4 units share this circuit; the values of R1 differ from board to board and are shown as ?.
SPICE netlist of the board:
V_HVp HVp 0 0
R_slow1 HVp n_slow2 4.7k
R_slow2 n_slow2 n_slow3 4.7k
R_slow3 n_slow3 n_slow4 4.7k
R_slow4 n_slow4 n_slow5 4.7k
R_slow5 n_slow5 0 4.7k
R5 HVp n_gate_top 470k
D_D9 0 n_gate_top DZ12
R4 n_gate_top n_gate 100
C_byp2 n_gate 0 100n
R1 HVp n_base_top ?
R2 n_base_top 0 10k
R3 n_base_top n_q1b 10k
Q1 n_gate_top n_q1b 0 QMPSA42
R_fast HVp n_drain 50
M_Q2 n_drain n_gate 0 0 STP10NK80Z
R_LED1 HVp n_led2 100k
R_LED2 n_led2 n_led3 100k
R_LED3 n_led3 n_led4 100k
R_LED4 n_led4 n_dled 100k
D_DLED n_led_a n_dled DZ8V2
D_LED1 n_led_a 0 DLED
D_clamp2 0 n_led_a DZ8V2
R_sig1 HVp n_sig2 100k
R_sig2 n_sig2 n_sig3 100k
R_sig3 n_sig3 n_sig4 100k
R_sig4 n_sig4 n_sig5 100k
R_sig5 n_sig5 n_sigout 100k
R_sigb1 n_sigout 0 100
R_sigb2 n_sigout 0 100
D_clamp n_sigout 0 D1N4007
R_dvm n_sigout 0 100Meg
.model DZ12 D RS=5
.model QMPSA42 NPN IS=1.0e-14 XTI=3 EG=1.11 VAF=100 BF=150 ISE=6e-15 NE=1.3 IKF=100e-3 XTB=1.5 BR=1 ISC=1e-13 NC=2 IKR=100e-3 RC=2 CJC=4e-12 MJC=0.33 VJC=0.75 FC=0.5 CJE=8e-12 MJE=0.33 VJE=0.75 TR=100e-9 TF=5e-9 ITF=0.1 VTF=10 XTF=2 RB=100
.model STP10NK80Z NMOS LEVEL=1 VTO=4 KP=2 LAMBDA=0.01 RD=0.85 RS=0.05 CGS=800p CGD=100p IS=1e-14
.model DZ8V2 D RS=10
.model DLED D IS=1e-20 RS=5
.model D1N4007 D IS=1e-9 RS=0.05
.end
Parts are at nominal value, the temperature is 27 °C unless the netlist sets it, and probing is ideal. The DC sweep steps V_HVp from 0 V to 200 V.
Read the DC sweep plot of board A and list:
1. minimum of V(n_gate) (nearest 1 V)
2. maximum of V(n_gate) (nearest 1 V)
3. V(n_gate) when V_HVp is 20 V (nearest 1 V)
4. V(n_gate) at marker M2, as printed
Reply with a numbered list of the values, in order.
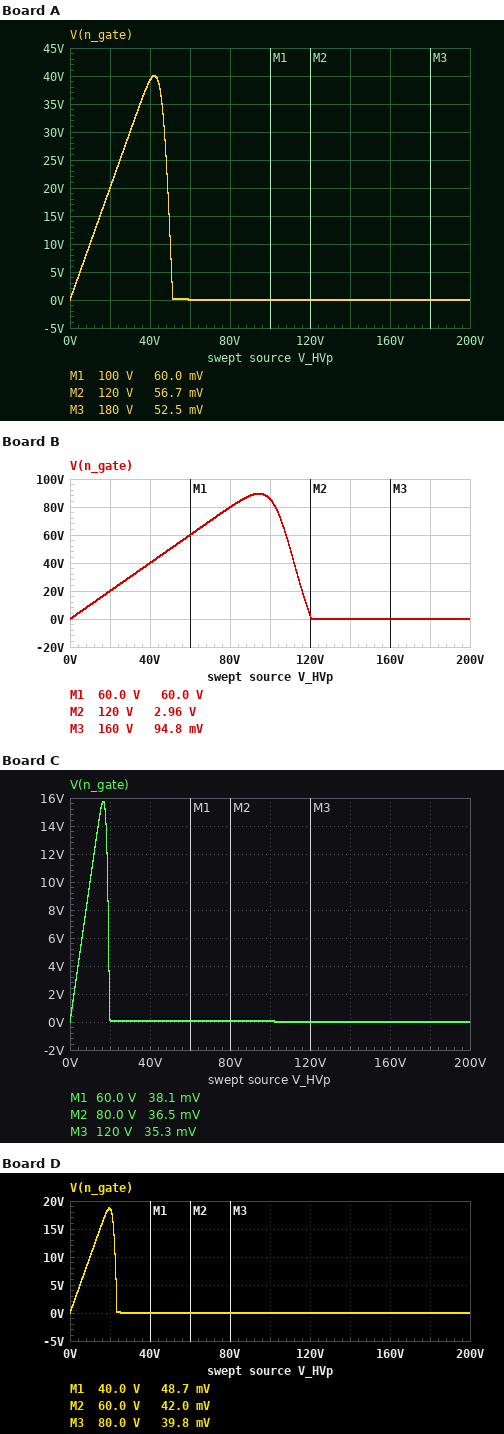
1. 0 V
2. 40 V
3. 20 V
4. 56.7 mV
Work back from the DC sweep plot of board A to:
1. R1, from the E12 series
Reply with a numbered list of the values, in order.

1. 820 kΩ
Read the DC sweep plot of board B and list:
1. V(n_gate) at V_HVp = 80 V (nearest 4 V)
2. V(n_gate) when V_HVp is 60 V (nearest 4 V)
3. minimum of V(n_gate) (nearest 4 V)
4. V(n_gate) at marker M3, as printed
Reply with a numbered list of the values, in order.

1. 80 V
2. 60 V
3. 0 V
4. 94.8 mV
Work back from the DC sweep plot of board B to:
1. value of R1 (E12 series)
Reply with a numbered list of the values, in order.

1. 1.8 MΩ
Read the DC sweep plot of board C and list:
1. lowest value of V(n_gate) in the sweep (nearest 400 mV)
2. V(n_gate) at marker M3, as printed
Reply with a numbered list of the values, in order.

1. 0 V
2. 35.3 mV
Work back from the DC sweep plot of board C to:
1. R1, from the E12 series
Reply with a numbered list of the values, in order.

1. 330 kΩ
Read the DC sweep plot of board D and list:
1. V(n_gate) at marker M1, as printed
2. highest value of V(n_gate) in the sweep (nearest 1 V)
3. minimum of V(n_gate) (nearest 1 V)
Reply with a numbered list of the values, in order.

1. 48.7 mV
2. 19 V
3. 0 V
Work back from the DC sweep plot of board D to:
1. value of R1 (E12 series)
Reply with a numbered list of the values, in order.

1. 390 kΩ
